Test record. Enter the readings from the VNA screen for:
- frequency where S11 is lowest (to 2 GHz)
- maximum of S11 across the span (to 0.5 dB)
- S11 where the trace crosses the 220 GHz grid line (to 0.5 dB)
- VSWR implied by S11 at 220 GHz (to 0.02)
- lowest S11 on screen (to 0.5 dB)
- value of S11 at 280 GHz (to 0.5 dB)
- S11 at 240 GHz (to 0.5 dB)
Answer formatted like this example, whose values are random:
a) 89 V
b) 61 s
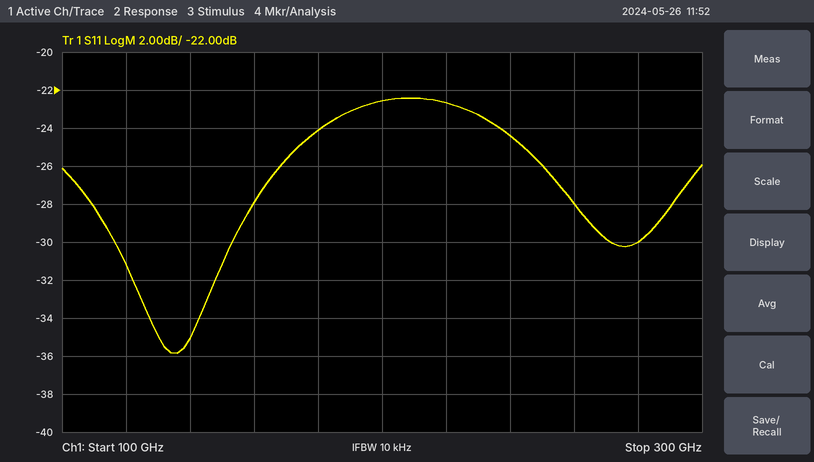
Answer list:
a) 136 GHz
b) -22.5 dB
c) -22.5 dB
d) 1.16
e) -36.0 dB
f) -30.0 dB
g) -24.5 dB
